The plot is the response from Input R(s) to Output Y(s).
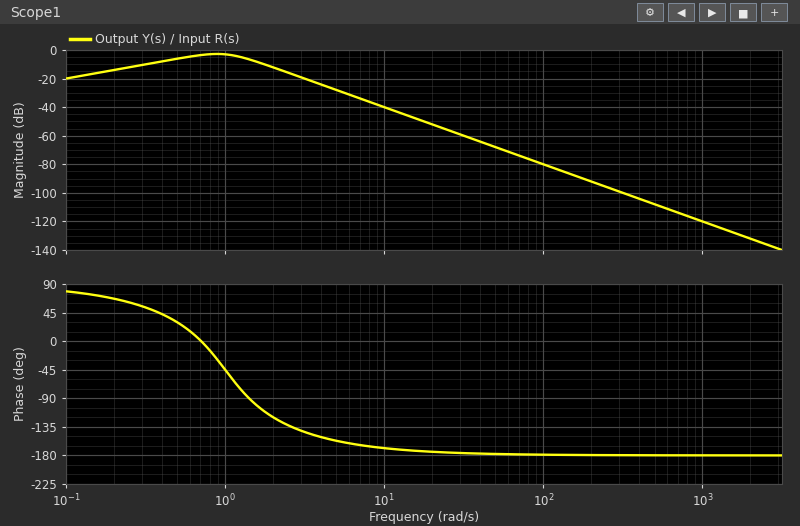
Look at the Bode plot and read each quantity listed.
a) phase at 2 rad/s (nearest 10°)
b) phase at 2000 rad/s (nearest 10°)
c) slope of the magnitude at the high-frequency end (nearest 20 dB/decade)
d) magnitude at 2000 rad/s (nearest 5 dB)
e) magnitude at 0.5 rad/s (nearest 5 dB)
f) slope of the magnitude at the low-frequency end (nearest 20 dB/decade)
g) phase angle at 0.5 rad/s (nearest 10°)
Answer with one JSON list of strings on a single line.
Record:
["-120°", "-180°", "-40 dB/decade", "-130 dB", "-5 dB", "20 dB/decade", "30°"]
